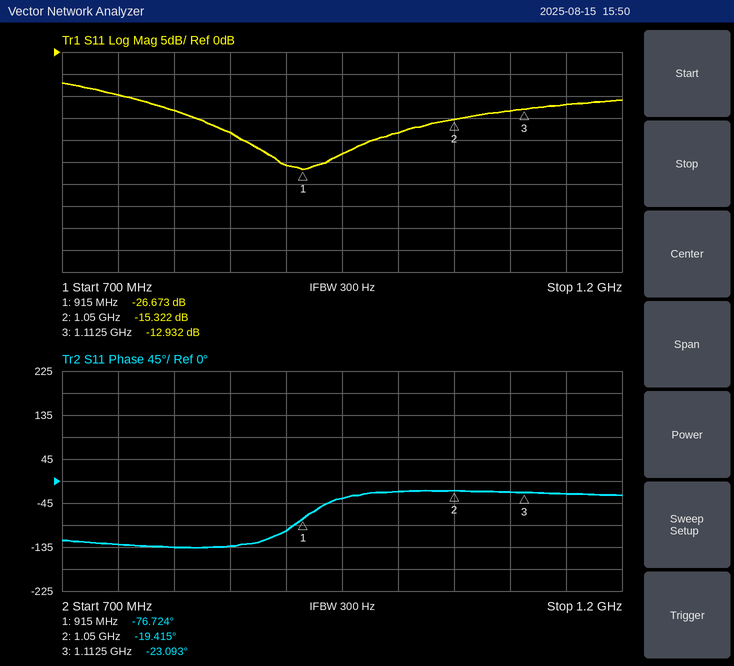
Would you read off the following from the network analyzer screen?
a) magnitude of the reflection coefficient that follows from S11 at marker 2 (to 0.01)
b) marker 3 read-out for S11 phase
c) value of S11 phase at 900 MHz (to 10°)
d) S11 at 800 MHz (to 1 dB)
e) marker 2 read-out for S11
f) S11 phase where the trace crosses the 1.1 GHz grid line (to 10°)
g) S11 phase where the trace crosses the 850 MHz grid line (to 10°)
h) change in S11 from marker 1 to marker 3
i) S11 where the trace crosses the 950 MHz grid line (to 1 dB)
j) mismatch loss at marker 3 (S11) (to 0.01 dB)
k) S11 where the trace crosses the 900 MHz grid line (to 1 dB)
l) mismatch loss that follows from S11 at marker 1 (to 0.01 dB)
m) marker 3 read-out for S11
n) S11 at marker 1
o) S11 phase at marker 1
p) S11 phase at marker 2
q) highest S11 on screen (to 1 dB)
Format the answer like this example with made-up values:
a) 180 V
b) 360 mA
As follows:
a) 0.17
b) -23.093°
c) -100°
d) -13 dB
e) -15.322 dB
f) -20°
g) -130°
h) 13.741 dB
i) -23 dB
j) 0.23 dB
k) -26 dB
l) 0.01 dB
m) -12.932 dB
n) -26.673 dB
o) -76.724°
p) -19.415°
q) -7 dB
